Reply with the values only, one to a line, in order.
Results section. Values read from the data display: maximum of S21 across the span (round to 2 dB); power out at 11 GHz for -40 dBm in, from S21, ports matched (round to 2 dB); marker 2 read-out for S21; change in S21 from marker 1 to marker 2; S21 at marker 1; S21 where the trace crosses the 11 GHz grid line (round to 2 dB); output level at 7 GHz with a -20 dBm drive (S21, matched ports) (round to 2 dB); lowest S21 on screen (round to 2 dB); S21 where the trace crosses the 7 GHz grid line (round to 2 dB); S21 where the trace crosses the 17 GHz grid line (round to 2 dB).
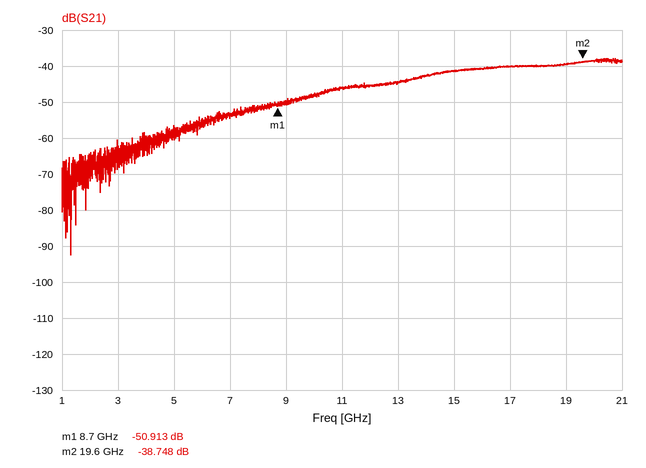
-38 dB
-86 dBm
-38.748 dB
12.165 dB
-50.913 dB
-46 dB
-74 dBm
-92 dB
-54 dB
-40 dB
